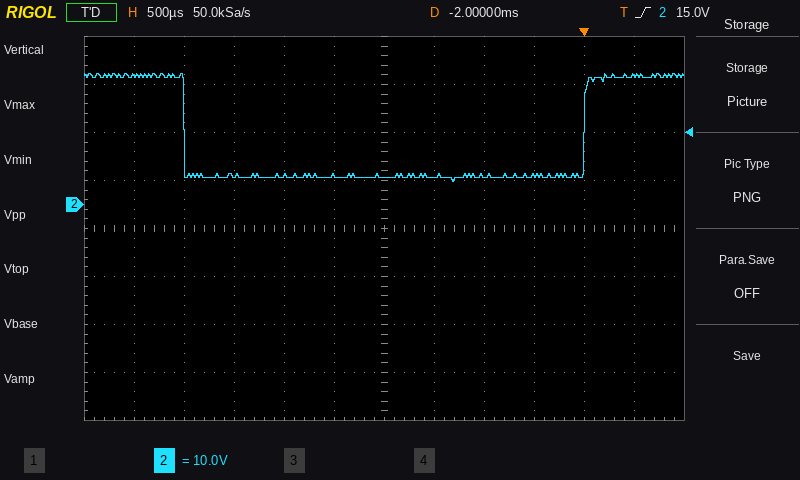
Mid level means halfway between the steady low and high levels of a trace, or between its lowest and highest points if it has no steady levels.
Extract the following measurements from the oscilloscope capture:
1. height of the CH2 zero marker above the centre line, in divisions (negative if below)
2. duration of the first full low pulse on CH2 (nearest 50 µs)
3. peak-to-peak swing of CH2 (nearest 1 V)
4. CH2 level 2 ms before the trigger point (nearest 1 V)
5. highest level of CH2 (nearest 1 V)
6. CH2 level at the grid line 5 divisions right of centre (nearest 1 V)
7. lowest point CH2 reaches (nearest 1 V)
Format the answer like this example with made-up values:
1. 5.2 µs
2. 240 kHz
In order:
1. +0.5 div
2. 4.00 ms
3. 22 V
4. 6 V
5. 27 V
6. 27 V
7. 5 V
